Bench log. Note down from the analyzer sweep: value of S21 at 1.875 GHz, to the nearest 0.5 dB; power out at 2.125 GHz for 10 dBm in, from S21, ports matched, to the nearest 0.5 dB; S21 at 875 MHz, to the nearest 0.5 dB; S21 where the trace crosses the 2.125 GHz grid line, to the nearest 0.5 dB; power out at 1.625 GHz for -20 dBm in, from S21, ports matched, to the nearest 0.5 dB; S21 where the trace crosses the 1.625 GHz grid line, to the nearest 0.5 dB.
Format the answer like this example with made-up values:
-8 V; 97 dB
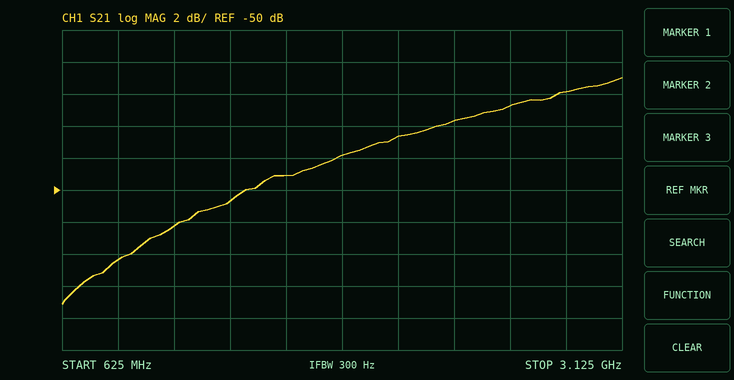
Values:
-48.0 dB; -36.5 dBm; -54.5 dB; -46.5 dB; -69.0 dBm; -49.0 dB
